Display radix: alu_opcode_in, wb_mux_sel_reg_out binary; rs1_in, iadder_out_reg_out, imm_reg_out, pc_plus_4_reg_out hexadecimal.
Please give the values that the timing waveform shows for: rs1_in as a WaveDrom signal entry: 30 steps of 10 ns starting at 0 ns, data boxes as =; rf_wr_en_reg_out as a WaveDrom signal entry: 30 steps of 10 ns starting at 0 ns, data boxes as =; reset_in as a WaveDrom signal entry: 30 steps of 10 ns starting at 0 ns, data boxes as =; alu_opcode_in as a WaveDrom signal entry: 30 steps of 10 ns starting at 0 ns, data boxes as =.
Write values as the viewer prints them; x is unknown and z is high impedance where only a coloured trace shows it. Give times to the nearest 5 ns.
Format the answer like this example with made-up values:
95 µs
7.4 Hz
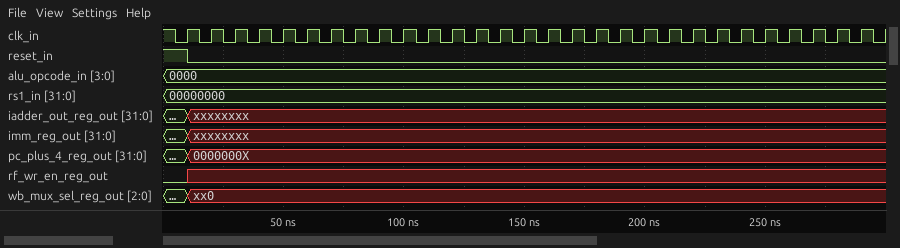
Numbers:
{name: 'rs1_in', wave: '=.............................', data: '00000000'}
{name: 'rf_wr_en_reg_out', wave: '0x............................'}
{name: 'reset_in', wave: '10............................'}
{name: 'alu_opcode_in', wave: '=.............................', data: '0000'}
